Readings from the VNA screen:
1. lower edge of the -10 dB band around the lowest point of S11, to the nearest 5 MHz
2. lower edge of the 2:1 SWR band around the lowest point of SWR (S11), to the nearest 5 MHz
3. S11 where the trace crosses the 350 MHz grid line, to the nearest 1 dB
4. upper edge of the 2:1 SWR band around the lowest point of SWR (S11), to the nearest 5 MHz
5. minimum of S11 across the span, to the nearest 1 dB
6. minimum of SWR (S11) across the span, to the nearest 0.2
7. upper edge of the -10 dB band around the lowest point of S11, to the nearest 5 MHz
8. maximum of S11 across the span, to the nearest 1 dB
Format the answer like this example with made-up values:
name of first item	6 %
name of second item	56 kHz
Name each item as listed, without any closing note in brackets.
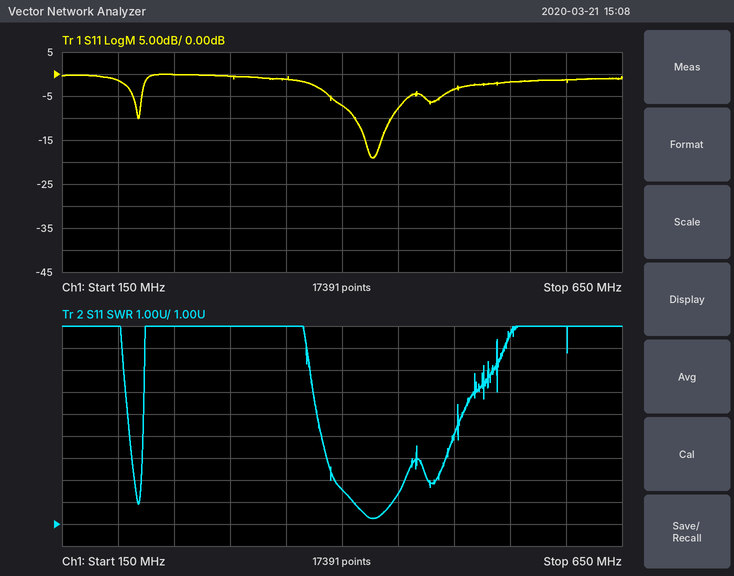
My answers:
lower edge of the -10 dB band around the lowest point of S11, to the nearest 5 MHz	410 MHz
lower edge of the 2:1 SWR band around the lowest point of SWR (S11), to the nearest 5 MHz	410 MHz
S11 where the trace crosses the 350 MHz grid line, to the nearest 1 dB	-1 dB
upper edge of the 2:1 SWR band around the lowest point of SWR (S11), to the nearest 5 MHz	445 MHz
minimum of S11 across the span, to the nearest 1 dB	-19 dB
minimum of SWR (S11) across the span, to the nearest 0.2	1.2
upper edge of the -10 dB band around the lowest point of S11, to the nearest 5 MHz	445 MHz
maximum of S11 across the span, to the nearest 1 dB	0 dB
